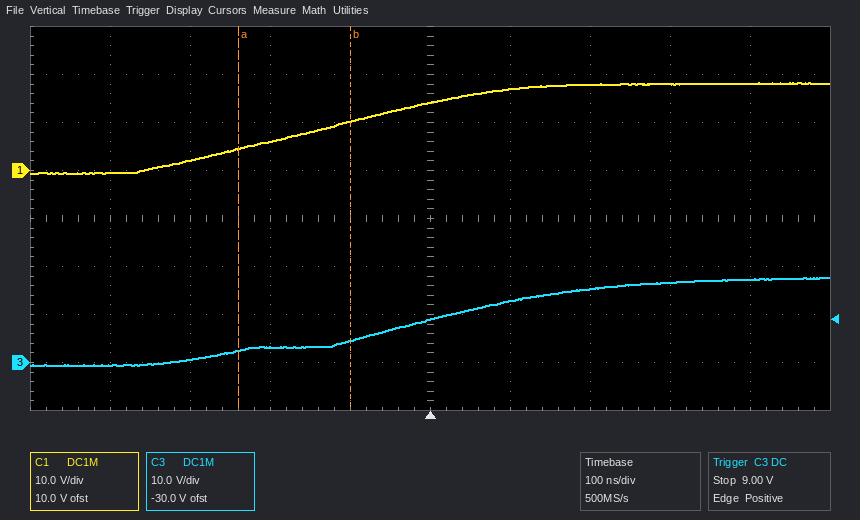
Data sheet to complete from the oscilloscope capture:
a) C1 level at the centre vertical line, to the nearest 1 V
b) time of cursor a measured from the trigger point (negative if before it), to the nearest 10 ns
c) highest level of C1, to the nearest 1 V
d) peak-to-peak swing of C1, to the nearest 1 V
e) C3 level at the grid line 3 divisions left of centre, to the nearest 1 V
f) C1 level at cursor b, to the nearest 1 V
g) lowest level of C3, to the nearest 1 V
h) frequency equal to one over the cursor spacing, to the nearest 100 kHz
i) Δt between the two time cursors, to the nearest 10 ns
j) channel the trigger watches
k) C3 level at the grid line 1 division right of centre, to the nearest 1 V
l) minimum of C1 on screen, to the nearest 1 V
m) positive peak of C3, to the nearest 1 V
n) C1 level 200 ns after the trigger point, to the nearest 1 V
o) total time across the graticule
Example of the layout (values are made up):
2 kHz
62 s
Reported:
14 V
-240 ns
18 V
19 V
1 V
10 V
-1 V
7.1 MHz
140 ns
C3
13 V
-1 V
18 V
18 V
1 µs
